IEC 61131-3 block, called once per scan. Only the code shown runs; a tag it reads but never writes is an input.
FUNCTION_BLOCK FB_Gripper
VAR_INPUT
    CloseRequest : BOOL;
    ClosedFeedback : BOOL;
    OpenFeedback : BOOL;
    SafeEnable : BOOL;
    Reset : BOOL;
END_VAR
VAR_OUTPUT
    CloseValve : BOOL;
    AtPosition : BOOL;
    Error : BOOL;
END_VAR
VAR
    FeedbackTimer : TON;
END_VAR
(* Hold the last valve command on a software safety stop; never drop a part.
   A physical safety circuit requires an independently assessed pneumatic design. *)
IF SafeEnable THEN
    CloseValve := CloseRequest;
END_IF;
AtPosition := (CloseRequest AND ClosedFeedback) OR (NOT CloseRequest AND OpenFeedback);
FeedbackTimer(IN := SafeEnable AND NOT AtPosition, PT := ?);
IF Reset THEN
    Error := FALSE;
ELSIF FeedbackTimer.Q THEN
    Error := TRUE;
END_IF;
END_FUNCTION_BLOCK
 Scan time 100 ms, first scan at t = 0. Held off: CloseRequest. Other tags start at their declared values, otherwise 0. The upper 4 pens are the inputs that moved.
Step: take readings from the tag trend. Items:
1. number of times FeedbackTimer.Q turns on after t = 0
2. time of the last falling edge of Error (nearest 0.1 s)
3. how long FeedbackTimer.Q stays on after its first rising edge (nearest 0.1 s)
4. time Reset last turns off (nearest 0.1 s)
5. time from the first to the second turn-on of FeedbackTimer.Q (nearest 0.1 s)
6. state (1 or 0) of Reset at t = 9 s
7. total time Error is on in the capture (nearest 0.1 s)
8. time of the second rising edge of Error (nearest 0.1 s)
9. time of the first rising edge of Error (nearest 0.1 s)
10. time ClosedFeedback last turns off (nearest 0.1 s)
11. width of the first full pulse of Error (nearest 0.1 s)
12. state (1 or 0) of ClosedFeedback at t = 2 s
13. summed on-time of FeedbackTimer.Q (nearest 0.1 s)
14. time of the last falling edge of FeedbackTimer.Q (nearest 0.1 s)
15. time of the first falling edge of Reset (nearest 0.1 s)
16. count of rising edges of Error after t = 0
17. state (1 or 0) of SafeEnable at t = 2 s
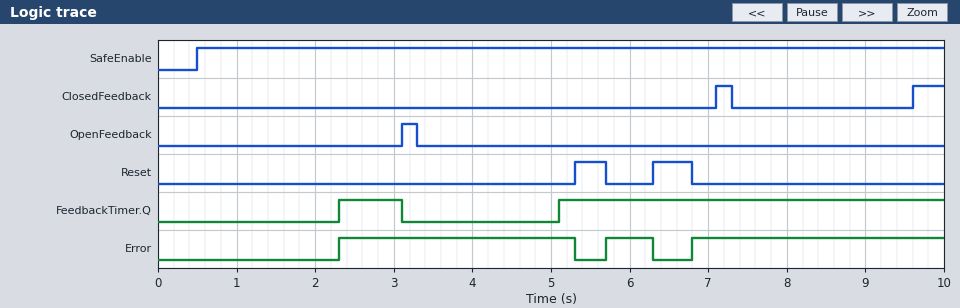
2
6.3 s
0.8 s
6.8 s
2.8 s
0
6.8 s
5.7 s
2.3 s
7.3 s
3.0 s
0
5.7 s
3.1 s
5.7 s
3
1
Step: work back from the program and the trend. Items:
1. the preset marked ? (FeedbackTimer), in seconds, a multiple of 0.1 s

1.8 s
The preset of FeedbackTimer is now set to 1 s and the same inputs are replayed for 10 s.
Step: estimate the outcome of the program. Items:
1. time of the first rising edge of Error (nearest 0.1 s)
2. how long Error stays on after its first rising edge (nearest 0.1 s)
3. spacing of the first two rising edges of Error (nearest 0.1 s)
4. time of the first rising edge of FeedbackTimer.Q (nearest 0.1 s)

1.5 s
3.8 s
4.2 s
1.5 s
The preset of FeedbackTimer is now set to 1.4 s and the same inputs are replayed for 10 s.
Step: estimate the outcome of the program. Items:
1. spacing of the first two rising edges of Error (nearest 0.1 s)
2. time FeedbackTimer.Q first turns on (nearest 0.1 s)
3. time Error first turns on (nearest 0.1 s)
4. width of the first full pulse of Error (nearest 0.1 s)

3.8 s
1.9 s
1.9 s
3.4 s
